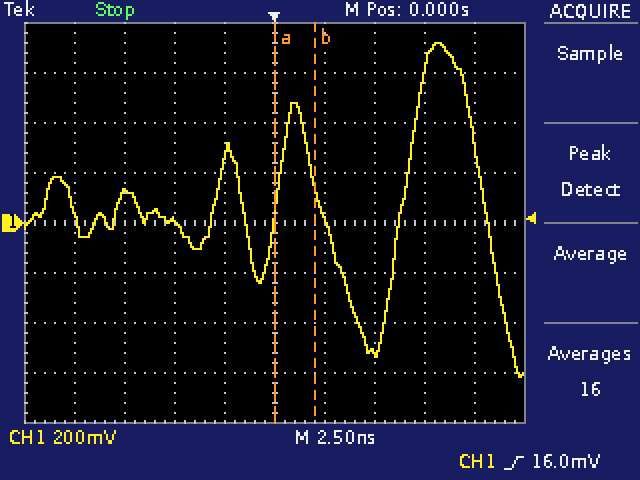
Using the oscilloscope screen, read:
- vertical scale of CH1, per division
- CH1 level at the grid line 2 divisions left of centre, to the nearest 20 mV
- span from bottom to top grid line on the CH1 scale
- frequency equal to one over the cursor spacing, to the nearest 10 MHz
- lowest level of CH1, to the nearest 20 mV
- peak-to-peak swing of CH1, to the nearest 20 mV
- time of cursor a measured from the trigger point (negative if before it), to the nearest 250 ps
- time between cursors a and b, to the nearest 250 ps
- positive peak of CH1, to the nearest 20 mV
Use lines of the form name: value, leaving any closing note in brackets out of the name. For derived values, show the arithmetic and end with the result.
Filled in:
vertical scale of CH1, per division: 200 mV
CH1 level at the grid line 2 divisions left of centre, to the nearest 20 mV: 0 mV
span from bottom to top grid line on the CH1 scale: 1.6 V
frequency equal to one over the cursor spacing, to the nearest 10 MHz: 1 / 2.00 ns ≈ 500 MHz
lowest level of CH1, to the nearest 20 mV: -620 mV
peak-to-peak swing of CH1, to the nearest 20 mV: 720 mV − (-620 mV) = 1.34 V
time of cursor a measured from the trigger point (negative if before it), to the nearest 250 ps: 0.00 ns
time between cursors a and b, to the nearest 250 ps: 2.00 ns
positive peak of CH1, to the nearest 20 mV: 720 mV
